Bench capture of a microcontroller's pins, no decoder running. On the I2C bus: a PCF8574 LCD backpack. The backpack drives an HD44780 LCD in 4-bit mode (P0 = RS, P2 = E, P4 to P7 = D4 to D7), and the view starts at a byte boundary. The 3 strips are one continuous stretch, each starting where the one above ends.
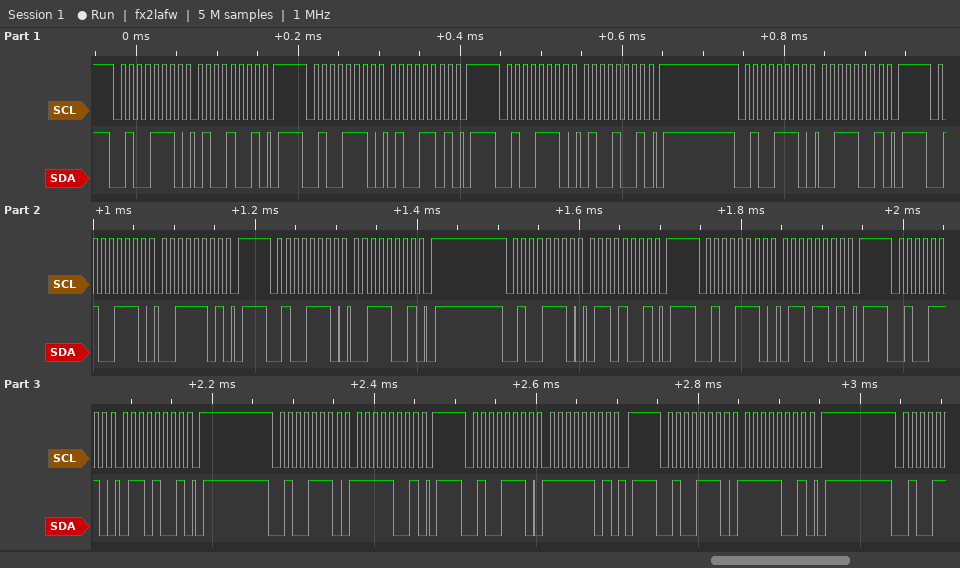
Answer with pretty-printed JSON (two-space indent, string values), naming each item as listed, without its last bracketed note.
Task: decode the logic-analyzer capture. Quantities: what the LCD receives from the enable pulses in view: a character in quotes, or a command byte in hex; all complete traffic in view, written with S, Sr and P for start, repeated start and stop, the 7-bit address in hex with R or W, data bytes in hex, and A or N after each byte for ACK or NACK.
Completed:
{
  "what the LCD receives from the enable pulses in view: a character in quotes, or a command byte in hex": "'C' 'o'",
  "all complete traffic in view, written with S, Sr and P for start, repeated start and stop, the 7-bit address in hex with R or W, data bytes in hex, and A or N after each byte for ACK or NACK": "S 27W A 49 A P S 27W A 4D A P S 27W A 49 A P S 27W A 39 A P S 27W A 3D A P S 27W A 39 A P S 27W A 69 A P S 27W A 6D A P S 27W A 69 A P S 27W A F9 A P S 27W A FD A P S 27W A F9 A P"
}
